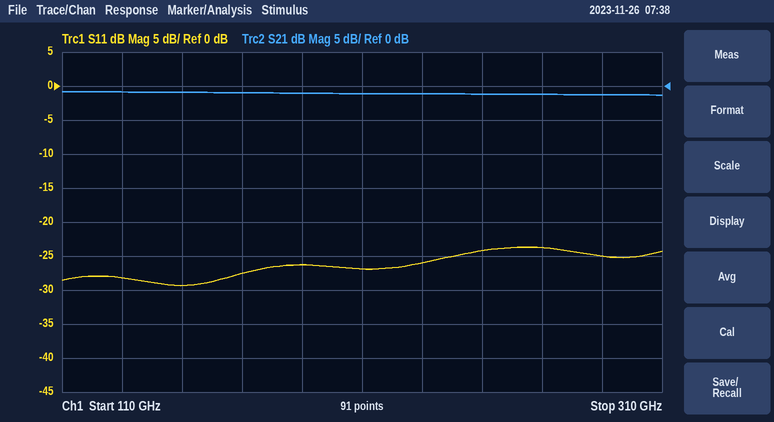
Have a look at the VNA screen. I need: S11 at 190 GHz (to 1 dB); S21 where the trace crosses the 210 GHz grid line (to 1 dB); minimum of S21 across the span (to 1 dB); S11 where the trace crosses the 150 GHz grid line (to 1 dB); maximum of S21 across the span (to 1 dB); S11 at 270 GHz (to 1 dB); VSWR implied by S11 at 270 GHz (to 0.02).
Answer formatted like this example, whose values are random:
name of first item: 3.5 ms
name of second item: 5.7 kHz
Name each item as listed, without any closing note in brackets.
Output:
S11 at 190 GHz: -26 dB
S21 where the trace crosses the 210 GHz grid line: -1 dB
minimum of S21 across the span: -1 dB
S11 where the trace crosses the 150 GHz grid line: -29 dB
maximum of S21 across the span: -1 dB
S11 at 270 GHz: -24 dB
VSWR implied by S11 at 270 GHz: 1.14
